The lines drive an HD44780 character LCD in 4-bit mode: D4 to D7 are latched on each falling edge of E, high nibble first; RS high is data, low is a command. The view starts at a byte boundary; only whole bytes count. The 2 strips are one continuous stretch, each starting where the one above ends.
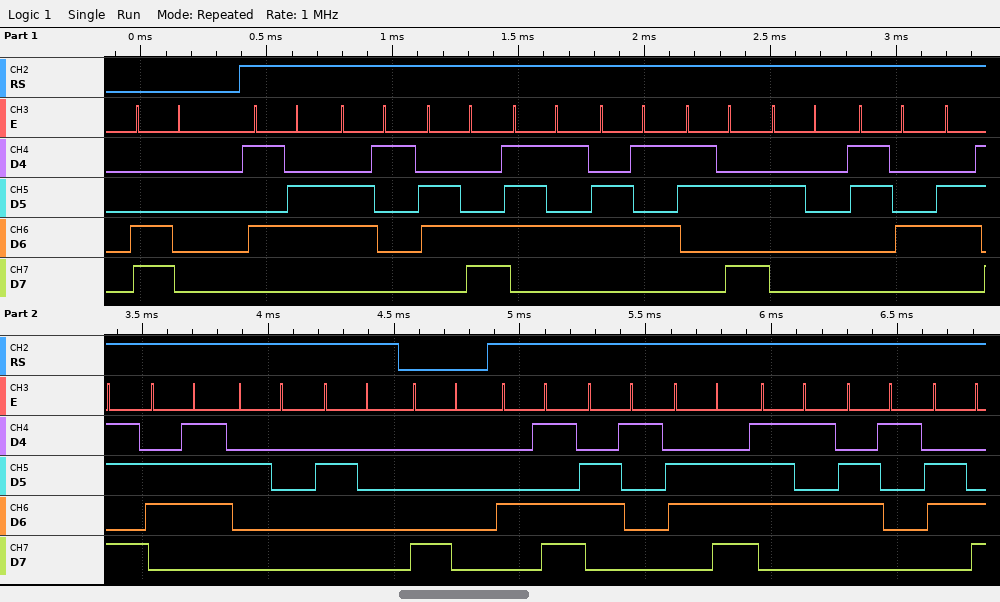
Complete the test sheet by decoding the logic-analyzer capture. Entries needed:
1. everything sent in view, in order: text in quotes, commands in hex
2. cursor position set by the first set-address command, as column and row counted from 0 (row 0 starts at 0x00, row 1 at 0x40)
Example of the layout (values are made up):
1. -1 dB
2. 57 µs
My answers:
1. 0xC0 "Value: 4kg  " 0x80 "Manual"
2. column 0, row 1
